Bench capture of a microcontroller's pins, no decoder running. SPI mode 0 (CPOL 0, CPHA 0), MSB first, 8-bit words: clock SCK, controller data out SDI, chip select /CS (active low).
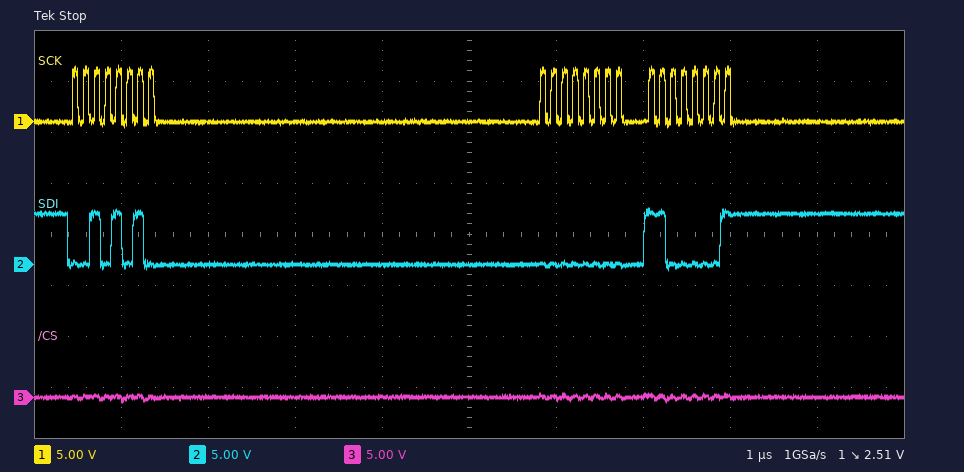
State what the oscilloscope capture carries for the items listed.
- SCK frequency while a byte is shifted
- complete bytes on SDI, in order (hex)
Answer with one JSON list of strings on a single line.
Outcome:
["8 MHz", "2A 00 C1"]
